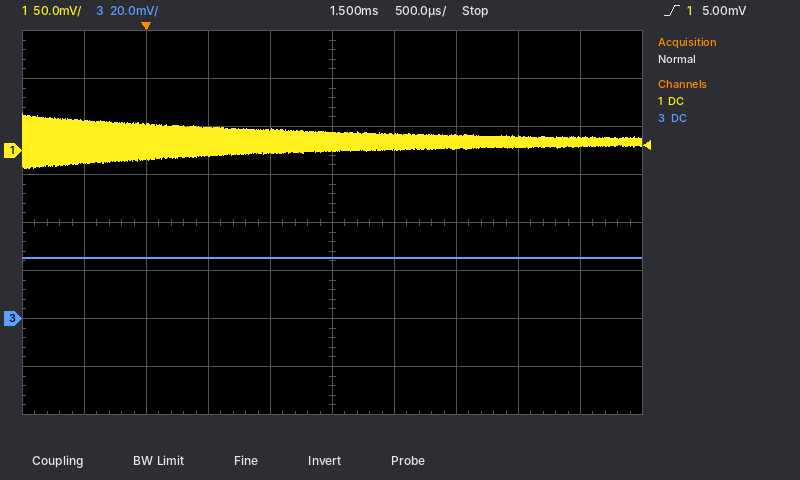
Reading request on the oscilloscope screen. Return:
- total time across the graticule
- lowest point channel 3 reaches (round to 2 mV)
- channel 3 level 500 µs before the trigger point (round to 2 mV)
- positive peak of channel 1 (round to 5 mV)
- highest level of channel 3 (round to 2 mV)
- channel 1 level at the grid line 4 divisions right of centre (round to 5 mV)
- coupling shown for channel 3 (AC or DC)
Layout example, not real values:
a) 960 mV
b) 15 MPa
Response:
a) 5 ms
b) 26 mV
c) 26 mV
d) 40 mV
e) 26 mV
f) 10 mV
g) DC
